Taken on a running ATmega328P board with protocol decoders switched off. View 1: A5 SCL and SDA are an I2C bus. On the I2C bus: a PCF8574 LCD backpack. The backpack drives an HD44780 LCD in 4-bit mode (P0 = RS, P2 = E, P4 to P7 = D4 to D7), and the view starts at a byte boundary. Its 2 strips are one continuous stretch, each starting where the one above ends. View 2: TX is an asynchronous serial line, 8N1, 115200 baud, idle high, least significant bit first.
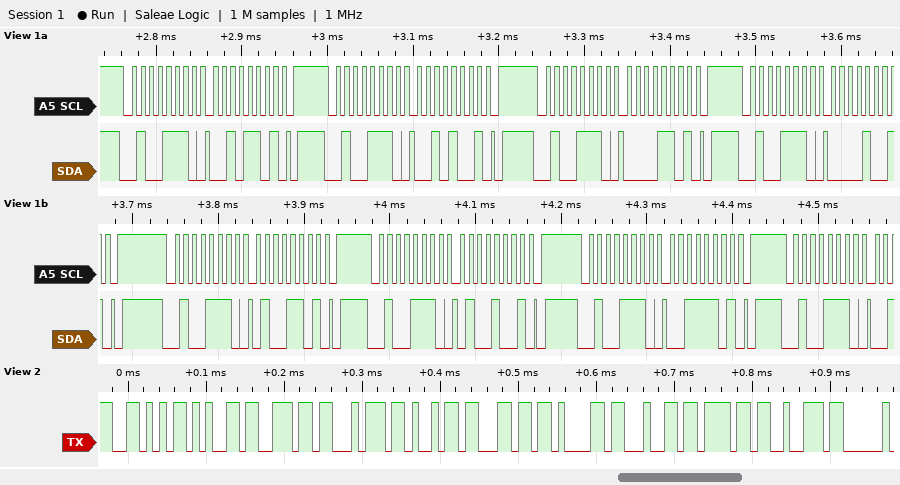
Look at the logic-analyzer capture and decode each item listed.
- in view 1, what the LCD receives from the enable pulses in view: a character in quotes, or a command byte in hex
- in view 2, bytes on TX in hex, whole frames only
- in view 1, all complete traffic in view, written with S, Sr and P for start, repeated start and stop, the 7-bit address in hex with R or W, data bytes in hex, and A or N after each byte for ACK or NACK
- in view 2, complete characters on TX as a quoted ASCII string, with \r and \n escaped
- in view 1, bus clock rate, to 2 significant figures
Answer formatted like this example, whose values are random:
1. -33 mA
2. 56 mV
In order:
1. ' '
2. 56 65 6E 74 69 6C 61 64 6F 72
3. S 27W A 2D A P S 27W A 29 A P S 27W A 0D A P S 27W A 09 A P S 27W A 4D A P S 27W A 49 A P S 27W A 3D A P S 27W A
4. "Ventilador"
5. 100 kHz
